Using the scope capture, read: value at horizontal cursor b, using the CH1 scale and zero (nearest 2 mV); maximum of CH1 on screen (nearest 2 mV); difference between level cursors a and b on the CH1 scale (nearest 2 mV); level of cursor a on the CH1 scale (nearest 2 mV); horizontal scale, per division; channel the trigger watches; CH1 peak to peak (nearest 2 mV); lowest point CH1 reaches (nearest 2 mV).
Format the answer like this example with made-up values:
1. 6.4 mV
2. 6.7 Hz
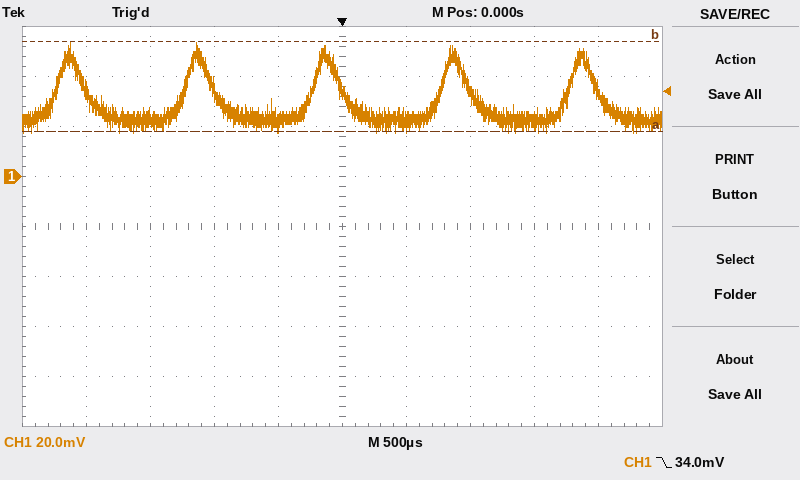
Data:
1. 54 mV
2. 54 mV
3. 36 mV
4. 18 mV
5. 500 µs
6. CH1
7. 36 mV
8. 18 mV
